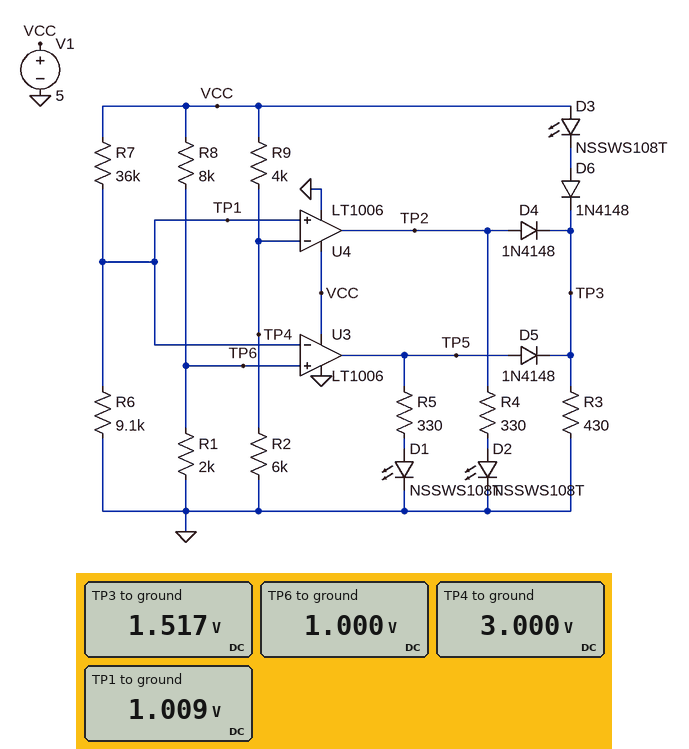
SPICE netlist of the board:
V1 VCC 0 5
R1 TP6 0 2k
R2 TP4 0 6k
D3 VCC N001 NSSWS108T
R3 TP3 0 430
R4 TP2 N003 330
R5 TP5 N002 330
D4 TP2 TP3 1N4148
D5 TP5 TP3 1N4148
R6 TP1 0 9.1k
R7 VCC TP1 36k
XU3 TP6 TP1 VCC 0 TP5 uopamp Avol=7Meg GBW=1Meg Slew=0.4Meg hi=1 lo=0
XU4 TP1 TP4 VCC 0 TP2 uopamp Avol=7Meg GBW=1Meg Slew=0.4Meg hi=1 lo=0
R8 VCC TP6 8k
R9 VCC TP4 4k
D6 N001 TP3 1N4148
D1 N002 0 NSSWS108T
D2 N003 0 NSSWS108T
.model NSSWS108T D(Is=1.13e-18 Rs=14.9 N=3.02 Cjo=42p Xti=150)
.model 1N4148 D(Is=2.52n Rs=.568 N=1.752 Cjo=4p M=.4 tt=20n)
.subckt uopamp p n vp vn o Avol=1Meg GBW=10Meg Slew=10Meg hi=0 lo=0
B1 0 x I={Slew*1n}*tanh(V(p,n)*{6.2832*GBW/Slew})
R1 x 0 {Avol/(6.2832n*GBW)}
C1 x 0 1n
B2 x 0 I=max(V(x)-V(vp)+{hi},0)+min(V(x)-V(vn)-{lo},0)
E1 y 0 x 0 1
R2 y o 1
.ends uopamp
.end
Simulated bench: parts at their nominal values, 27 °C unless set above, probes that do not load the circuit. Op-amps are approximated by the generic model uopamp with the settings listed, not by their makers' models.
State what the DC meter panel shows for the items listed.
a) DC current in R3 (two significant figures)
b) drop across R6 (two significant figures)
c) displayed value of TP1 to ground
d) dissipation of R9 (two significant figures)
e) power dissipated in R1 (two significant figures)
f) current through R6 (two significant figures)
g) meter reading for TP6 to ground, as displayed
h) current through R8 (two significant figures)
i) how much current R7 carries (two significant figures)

3.5 mA
1.0 V
1.009 V
1.0 mW
500 µW
110 µA
1.000 V
500 µA
110 µA
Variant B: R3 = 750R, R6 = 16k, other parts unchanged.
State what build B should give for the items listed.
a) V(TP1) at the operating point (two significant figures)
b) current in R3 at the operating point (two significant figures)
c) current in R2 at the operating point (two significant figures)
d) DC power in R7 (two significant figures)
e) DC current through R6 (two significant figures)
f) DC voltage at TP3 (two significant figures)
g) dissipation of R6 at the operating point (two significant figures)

1.5 V
2.1 mA
500 µA
330 µW
96 µA
1.6 V
150 µW
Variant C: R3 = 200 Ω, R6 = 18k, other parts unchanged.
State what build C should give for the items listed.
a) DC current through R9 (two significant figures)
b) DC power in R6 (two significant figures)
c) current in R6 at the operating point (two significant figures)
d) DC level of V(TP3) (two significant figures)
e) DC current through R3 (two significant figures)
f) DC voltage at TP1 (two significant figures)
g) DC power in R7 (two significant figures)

500 µA
150 µW
93 µA
1.4 V
6.9 mA
1.7 V
310 µW
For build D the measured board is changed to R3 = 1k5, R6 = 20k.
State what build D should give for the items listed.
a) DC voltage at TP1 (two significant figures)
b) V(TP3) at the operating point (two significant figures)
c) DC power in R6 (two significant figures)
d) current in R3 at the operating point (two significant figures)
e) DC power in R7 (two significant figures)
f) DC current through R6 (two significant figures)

1.8 V
1.7 V
160 µW
1.1 mA
290 µW
89 µA
